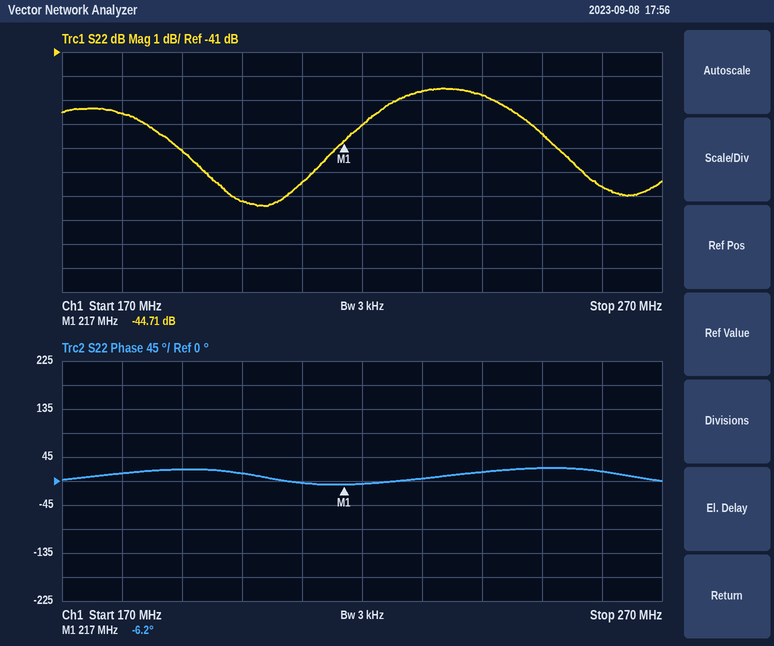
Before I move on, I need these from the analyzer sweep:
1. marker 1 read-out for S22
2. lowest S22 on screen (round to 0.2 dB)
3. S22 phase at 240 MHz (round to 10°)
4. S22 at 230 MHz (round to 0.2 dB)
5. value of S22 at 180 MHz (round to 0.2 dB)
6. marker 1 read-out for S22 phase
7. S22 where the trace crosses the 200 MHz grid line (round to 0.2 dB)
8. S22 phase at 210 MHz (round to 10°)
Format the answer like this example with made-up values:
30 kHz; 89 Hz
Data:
-44.71 dB; -47.4 dB; 20°; -42.6 dB; -43.6 dB; -6.2°; -47.2 dB; 0°
